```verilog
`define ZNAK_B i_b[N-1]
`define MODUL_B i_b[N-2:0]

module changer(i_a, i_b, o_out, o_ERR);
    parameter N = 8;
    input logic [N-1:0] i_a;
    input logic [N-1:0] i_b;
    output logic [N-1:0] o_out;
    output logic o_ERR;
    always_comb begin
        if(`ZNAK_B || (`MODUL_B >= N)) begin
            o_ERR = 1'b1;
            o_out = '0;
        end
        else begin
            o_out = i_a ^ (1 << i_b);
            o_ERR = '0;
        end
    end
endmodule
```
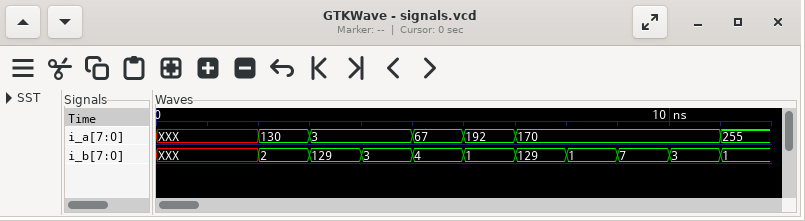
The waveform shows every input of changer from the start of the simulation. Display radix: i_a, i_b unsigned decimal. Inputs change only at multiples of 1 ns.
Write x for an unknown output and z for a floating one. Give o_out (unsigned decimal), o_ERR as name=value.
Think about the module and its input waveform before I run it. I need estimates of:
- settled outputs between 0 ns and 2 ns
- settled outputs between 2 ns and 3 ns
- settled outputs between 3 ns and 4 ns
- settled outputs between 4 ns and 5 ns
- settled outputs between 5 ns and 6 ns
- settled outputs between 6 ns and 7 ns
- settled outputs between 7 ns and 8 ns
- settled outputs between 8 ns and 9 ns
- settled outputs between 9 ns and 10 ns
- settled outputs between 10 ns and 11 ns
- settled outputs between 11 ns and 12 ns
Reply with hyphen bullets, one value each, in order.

- o_out=x, o_ERR=0
- o_out=134, o_ERR=0
- o_out=0, o_ERR=1
- o_out=11, o_ERR=0
- o_out=83, o_ERR=0
- o_out=194, o_ERR=0
- o_out=0, o_ERR=1
- o_out=168, o_ERR=0
- o_out=42, o_ERR=0
- o_out=162, o_ERR=0
- o_out=253, o_ERR=0
